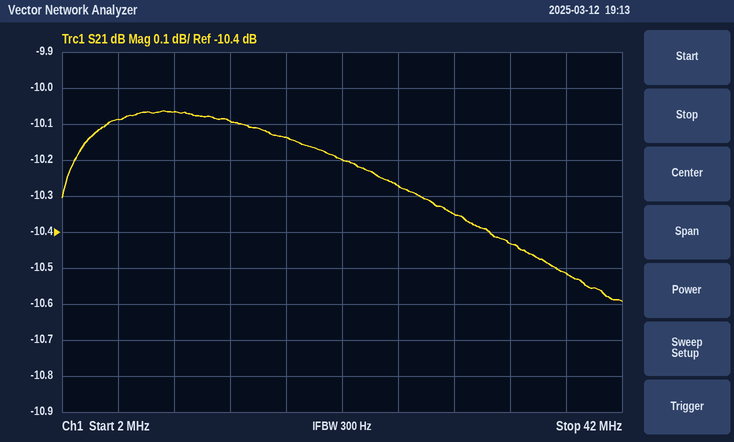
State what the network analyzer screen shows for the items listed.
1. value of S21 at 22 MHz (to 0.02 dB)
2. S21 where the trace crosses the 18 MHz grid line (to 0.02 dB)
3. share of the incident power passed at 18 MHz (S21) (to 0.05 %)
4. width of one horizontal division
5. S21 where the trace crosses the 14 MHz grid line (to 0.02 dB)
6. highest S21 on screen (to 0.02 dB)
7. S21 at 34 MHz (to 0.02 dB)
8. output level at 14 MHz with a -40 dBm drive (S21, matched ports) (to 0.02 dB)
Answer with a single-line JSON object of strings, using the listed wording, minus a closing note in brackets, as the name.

{"value of S21 at 22 MHz": "-10.20 dB", "S21 where the trace crosses the 18 MHz grid line": "-10.14 dB", "share of the incident power passed at 18 MHz (S21)": "9.70 %", "width of one horizontal division": "4 MHz", "S21 where the trace crosses the 14 MHz grid line": "-10.10 dB", "highest S21 on screen": "-10.06 dB", "S21 at 34 MHz": "-10.44 dB", "output level at 14 MHz with a -40 dBm drive (S21, matched ports)": "-50.10 dBm"}
